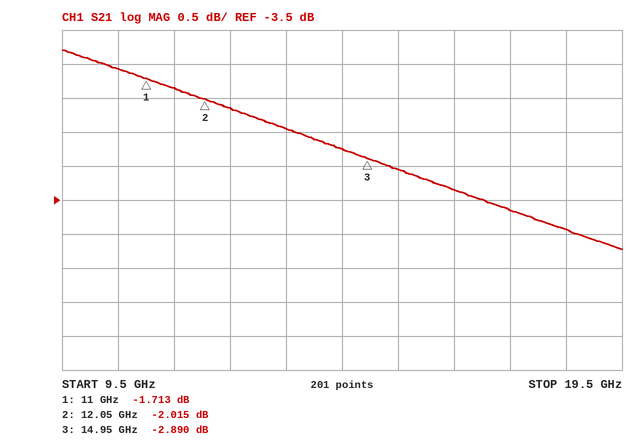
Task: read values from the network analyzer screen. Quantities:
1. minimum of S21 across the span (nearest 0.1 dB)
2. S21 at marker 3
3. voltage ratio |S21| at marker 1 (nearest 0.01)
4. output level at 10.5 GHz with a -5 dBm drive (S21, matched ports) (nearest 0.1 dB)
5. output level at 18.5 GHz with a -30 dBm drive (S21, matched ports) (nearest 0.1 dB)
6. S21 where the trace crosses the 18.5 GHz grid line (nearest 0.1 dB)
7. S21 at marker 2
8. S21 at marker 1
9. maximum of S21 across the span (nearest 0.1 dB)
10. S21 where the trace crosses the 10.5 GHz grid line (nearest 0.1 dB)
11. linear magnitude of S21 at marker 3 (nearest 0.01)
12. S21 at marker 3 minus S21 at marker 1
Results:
-4.2 dB
-2.890 dB
0.82
-6.6 dBm
-33.9 dBm
-3.9 dB
-2.015 dB
-1.713 dB
-1.3 dB
-1.6 dB
0.72
-1.177 dB
